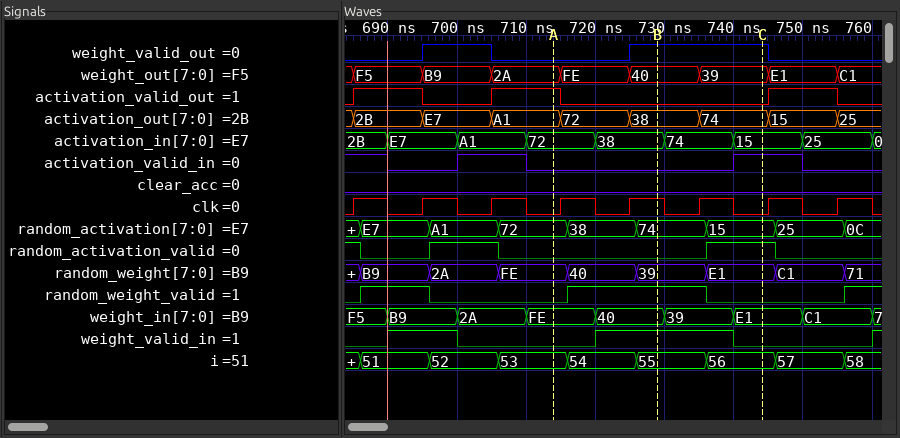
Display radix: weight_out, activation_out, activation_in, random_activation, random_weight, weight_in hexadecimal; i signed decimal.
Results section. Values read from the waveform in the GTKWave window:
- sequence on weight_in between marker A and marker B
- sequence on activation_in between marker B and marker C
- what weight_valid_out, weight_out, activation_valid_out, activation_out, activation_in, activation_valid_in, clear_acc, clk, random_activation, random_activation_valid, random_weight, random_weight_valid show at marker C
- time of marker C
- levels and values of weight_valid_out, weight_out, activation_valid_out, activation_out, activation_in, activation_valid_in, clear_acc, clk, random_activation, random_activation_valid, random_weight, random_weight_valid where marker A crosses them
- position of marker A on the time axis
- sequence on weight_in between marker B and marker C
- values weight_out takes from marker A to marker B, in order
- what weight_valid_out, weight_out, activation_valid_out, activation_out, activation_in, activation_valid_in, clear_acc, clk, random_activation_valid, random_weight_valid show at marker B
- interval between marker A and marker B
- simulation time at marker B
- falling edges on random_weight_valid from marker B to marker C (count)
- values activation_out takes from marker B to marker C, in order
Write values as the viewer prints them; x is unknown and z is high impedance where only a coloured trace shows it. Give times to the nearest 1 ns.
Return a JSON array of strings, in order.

["FE, 40", "38, 74, 15", "weight_valid_out=1, weight_out=39, activation_valid_out=0, activation_out=74, activation_in=15, activation_valid_in=1, clear_acc=0, clk=0, random_activation=15, random_activation_valid=1, random_weight=E1, random_weight_valid=0", "744 ns", "weight_valid_out=0, weight_out=2A, activation_valid_out=1, activation_out=A1, activation_in=72, activation_valid_in=0, clear_acc=0, clk=0, random_activation=72, random_activation_valid=0, random_weight=FE, random_weight_valid=0", "714 ns", "40, 39, E1", "2A, FE, 40", "weight_valid_out=1, weight_out=40, activation_valid_out=0, activation_out=38, activation_in=38, activation_valid_in=0, clear_acc=0, clk=1, random_activation_valid=0, random_weight_valid=1", "15 ns", "729 ns", "1", "38, 74"]
